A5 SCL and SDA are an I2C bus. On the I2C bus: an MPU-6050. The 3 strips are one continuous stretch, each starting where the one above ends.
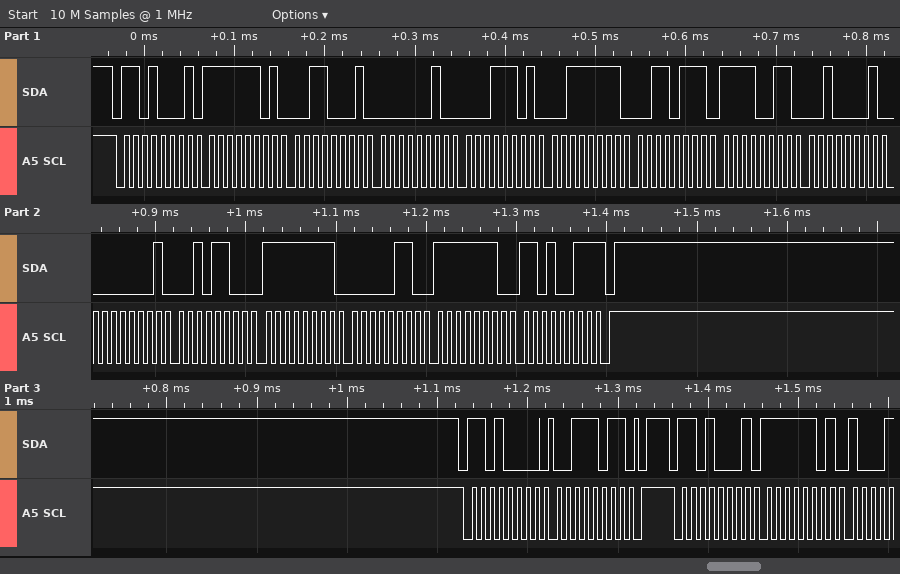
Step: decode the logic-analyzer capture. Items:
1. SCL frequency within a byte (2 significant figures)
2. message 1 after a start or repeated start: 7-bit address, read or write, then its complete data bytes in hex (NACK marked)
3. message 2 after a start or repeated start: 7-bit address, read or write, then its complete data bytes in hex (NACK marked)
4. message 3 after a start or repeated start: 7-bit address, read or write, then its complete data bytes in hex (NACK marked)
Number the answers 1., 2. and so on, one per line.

1. 100 kHz
2. 0x68 read: FD 31 02 1D 3F 37 F3 21 01 2C FF 06 FE D3 NACK
3. 0x68 write: 3B
4. 0x68 read: FD
